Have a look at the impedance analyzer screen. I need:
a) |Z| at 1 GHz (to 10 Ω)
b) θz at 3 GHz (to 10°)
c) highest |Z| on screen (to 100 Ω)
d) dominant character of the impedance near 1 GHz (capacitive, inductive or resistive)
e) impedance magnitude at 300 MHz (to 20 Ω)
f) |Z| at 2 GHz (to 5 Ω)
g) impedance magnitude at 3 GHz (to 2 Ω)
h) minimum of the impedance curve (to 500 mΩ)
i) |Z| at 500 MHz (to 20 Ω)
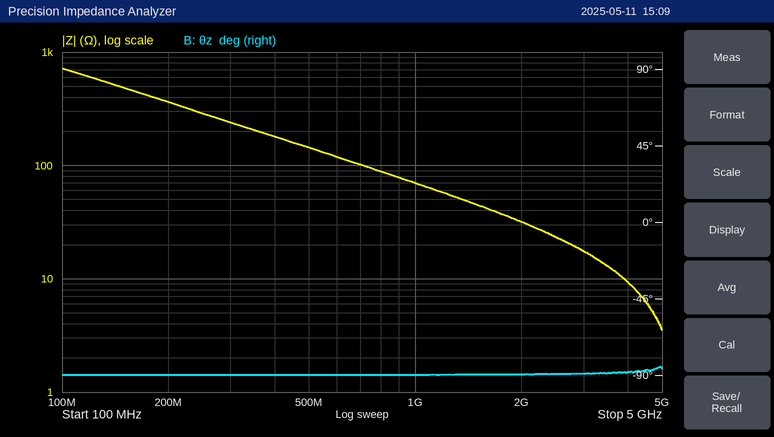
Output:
70 Ω
-90°
700 Ω
capacitive
240 Ω
30 Ω
18 Ω
3.5 Ω
140 Ω
